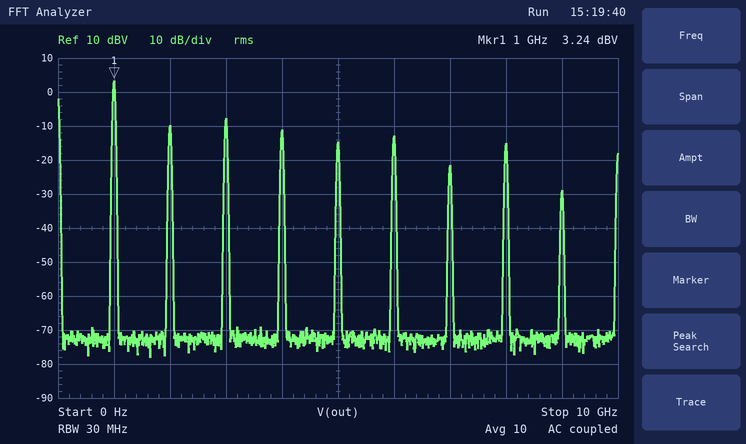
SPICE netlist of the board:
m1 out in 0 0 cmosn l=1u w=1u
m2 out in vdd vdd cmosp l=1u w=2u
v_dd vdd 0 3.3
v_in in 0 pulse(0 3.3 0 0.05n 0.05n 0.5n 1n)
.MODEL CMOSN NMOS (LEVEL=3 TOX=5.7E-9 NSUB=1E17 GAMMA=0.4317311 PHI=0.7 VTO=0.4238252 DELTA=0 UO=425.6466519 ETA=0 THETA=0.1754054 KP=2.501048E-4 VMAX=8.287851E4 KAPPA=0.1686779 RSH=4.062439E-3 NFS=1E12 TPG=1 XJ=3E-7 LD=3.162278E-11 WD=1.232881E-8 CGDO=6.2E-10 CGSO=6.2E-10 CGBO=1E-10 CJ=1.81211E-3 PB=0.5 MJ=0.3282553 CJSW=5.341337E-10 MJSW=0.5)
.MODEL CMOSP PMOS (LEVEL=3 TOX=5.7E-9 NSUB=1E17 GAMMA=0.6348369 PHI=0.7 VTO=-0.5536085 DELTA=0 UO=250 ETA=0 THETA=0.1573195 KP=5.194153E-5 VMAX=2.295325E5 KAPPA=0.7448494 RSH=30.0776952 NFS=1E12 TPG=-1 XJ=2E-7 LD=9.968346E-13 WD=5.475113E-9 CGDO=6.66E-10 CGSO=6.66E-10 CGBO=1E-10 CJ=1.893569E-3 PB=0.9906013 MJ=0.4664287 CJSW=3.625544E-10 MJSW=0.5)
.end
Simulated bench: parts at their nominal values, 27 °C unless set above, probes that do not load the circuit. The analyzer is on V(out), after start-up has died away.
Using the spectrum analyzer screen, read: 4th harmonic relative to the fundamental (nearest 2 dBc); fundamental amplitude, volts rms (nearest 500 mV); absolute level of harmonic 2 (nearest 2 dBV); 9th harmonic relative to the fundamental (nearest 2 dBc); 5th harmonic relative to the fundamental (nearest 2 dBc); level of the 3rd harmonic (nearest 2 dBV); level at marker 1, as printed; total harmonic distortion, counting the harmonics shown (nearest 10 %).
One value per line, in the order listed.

-14 dBc
1.5 V
-10 dBV
-32 dBc
-18 dBc
-8 dBV
3.24 dBV
50 %
